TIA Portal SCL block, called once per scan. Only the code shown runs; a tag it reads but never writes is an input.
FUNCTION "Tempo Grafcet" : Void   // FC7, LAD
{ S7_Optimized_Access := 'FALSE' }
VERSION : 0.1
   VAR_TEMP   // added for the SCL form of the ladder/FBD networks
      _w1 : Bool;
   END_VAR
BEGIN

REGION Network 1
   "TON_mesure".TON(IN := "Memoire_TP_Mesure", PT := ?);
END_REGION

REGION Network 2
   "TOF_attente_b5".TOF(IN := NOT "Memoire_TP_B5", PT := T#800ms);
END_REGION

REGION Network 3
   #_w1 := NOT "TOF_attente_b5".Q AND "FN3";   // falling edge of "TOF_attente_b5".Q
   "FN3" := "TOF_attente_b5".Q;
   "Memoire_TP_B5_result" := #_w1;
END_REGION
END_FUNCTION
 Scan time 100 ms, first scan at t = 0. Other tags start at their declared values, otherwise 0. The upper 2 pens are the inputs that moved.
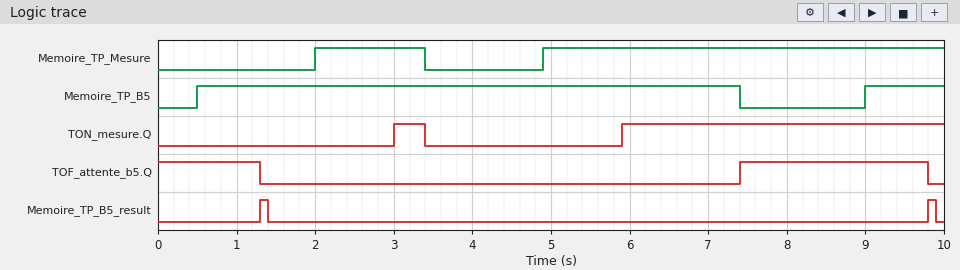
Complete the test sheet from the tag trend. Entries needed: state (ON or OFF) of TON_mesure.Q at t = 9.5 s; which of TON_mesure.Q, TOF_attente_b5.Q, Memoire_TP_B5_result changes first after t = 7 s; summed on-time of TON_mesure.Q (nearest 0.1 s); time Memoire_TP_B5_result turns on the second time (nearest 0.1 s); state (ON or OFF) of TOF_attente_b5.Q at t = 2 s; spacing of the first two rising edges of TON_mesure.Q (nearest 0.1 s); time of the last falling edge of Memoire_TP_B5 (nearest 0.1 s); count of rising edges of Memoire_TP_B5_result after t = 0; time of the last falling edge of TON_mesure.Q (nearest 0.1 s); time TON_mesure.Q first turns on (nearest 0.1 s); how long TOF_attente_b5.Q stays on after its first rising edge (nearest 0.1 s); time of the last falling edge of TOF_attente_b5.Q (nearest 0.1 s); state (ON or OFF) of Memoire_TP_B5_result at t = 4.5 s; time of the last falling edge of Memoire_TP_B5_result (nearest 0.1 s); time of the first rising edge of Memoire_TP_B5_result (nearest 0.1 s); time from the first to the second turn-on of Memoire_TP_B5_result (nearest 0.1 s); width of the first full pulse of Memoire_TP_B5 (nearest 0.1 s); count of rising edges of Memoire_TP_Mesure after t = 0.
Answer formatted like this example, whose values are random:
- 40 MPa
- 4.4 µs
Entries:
- ON
- TOF_attente_b5.Q
- 4.5 s
- 9.8 s
- OFF
- 2.9 s
- 7.4 s
- 2
- 3.4 s
- 3.0 s
- 2.4 s
- 9.8 s
- OFF
- 9.9 s
- 1.3 s
- 8.5 s
- 6.9 s
- 2
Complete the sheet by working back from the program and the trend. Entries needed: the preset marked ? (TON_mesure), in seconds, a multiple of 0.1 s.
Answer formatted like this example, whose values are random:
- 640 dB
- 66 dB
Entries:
- 1.0 s
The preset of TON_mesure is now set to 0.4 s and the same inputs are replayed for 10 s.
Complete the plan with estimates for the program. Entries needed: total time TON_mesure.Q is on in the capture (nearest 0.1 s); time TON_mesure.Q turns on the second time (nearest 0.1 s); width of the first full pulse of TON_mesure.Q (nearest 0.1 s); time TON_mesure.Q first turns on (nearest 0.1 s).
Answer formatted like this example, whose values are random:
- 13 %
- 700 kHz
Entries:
- 5.7 s
- 5.3 s
- 1.0 s
- 2.4 s
